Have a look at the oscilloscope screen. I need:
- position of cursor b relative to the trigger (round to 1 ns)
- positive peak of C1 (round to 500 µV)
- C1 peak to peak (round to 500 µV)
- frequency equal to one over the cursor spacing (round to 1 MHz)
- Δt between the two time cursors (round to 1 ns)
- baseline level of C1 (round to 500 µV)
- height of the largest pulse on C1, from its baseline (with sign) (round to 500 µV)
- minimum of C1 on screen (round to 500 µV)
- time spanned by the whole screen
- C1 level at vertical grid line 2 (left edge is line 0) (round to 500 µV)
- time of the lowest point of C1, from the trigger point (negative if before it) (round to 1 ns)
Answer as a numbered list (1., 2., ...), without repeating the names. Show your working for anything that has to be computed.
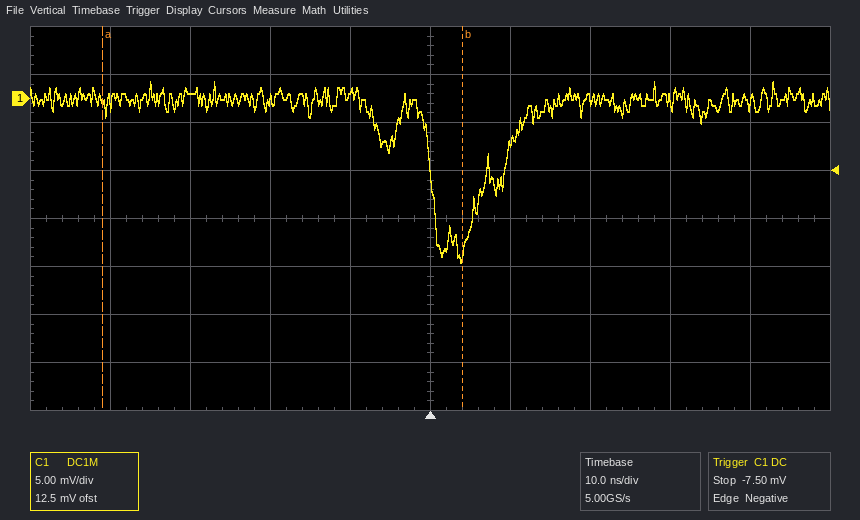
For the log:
1. +4 ns
2. 2.0 mV
3. 2.0 mV − (-17.0 mV) = 19.0 mV
4. 1 / 45 ns ≈ 22 MHz
5. 45 ns
6. 0.0 mV
7. -17.0 mV − (0.0 mV) = -17.0 mV
8. -17.0 mV
9. 100 ns
10. 1.0 mV
11. +4 ns
